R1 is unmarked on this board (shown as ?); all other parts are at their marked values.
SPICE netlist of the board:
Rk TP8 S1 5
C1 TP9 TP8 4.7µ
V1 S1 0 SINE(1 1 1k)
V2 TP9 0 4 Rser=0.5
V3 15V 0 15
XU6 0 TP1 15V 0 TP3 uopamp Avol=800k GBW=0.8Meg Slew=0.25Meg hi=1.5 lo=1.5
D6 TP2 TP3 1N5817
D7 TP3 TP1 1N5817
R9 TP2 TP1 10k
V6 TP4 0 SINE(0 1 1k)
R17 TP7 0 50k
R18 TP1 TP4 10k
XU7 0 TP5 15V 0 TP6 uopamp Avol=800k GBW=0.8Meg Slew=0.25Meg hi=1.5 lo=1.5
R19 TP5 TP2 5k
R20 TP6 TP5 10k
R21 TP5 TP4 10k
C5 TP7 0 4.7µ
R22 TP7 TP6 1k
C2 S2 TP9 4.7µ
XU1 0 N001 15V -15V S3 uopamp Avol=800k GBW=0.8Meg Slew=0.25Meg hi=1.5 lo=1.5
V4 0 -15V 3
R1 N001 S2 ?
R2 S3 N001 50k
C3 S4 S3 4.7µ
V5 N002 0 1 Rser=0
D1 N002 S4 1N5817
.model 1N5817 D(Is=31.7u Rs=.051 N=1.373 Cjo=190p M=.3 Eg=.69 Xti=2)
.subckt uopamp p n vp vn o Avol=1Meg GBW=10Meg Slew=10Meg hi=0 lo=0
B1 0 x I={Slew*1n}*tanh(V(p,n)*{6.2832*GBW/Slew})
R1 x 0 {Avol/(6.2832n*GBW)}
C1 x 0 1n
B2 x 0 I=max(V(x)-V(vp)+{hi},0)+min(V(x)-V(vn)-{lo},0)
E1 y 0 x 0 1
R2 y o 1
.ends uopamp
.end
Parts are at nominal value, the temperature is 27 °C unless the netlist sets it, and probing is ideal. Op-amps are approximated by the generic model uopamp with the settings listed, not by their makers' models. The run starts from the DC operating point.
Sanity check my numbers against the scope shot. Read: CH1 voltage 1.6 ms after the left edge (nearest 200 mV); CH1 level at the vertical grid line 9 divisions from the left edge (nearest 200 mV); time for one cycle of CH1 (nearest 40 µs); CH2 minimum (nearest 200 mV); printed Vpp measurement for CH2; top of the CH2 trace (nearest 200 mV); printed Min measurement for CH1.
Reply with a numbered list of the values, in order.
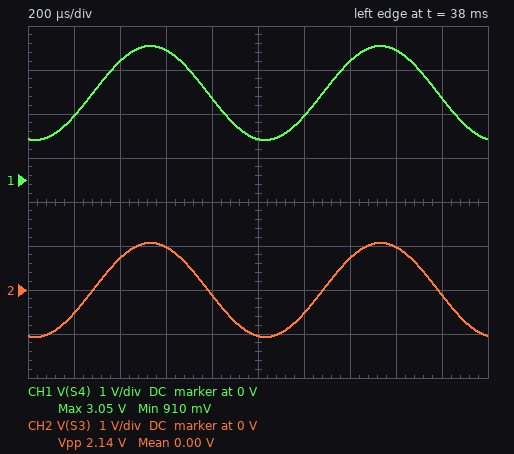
1. 3.0 V
2. 1.8 V
3. 1.00 ms
4. -1.0 V
5. 2.14 V
6. 1.0 V
7. 910 mV
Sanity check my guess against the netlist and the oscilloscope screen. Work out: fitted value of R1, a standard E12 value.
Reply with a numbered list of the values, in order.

1. 680 Ω
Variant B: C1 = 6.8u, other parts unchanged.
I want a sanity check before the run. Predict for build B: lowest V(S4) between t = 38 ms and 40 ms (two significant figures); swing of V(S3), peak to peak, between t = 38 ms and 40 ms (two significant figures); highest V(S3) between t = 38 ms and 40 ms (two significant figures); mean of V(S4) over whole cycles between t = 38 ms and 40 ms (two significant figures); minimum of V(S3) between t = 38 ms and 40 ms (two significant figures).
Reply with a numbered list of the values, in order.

1. 910 mV
2. 3.0 V
3. 1.5 V
4. 2.4 V
5. -1.5 V
